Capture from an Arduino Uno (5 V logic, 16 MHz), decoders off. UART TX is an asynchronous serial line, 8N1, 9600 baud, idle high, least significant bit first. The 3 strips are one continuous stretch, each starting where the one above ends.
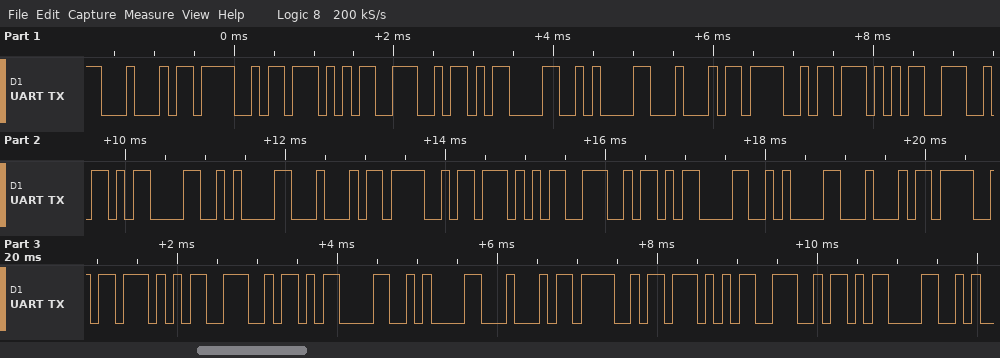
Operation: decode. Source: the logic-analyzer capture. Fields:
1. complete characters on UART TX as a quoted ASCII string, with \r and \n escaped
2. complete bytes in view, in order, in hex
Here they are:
"DOWN\r\nDOWN\r\nDOWN\r\nDOWN\r\nDOWN\r"
44 4F 57 4E 0D 0A 44 4F 57 4E 0D 0A 44 4F 57 4E 0D 0A 44 4F 57 4E 0D 0A 44 4F 57 4E 0D
